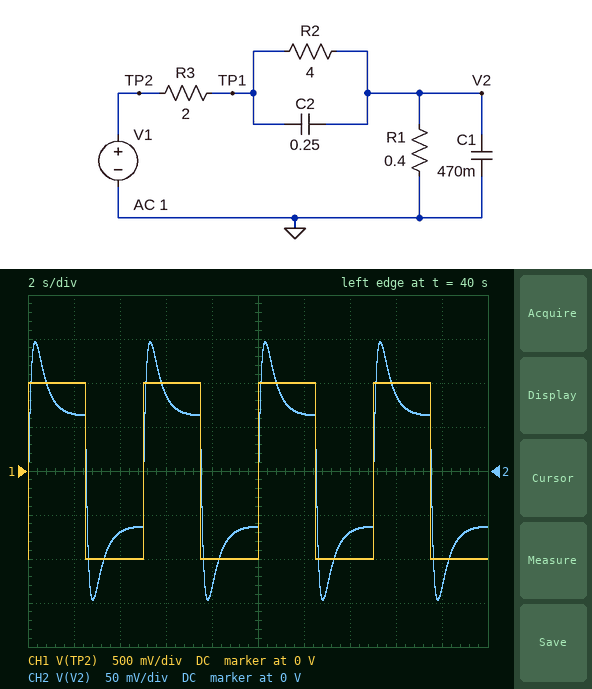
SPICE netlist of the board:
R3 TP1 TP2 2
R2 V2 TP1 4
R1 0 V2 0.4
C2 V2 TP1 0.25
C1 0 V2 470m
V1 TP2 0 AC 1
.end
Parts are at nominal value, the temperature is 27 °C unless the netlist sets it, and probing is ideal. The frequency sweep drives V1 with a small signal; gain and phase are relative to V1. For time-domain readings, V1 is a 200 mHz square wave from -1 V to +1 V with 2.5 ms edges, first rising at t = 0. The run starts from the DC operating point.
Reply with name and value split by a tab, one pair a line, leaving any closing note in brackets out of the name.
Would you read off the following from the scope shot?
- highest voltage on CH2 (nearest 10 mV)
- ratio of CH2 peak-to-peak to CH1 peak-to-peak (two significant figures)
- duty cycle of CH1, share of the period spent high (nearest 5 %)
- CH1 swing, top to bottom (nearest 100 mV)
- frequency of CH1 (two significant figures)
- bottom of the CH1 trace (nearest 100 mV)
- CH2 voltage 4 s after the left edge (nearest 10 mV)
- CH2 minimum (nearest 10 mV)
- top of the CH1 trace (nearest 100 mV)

highest voltage on CH2	150 mV
ratio of CH2 peak-to-peak to CH1 peak-to-peak	0.15
duty cycle of CH1, share of the period spent high	50 %
CH1 swing, top to bottom	2.0 V
frequency of CH1	200 mHz
bottom of the CH1 trace	-1.0 V
CH2 voltage 4 s after the left edge	-70 mV
CH2 minimum	-150 mV
top of the CH1 trace	1.0 V
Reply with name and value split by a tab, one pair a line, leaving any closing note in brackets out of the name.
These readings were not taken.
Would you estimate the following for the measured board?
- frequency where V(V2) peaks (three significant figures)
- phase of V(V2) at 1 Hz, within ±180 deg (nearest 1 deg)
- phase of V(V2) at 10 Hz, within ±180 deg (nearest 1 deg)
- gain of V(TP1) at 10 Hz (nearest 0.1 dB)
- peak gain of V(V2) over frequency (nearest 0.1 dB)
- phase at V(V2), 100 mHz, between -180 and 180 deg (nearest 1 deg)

frequency where V(V2) peaks	604 mHz
phase of V(V2) at 1 Hz, within ±180 deg	-30 deg
phase of V(V2) at 10 Hz, within ±180 deg	-82 deg
gain of V(TP1) at 10 Hz	-26.3 dB
peak gain of V(V2) over frequency	-18.6 dB
phase at V(V2), 100 mHz, between -180 and 180 deg	13 deg
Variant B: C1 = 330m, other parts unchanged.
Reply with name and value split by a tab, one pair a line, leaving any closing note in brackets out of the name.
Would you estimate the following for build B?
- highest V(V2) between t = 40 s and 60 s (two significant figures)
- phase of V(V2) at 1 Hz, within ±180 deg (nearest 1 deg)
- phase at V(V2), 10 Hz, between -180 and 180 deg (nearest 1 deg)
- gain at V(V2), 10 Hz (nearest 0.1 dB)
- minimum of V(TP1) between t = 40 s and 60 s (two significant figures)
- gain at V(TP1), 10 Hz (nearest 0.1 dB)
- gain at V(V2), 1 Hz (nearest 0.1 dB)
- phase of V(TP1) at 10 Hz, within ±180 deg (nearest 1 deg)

highest V(V2) between t = 40 s and 60 s	170 mV
phase of V(V2) at 1 Hz, within ±180 deg	-20 deg
phase at V(V2), 10 Hz, between -180 and 180 deg	-80 deg
gain at V(V2), 10 Hz	-32.5 dB
minimum of V(TP1) between t = 40 s and 60 s	-690 mV
gain at V(TP1), 10 Hz	-25.1 dB
gain at V(V2), 1 Hz	-18.1 dB
phase of V(TP1) at 10 Hz, within ±180 deg	-83 deg
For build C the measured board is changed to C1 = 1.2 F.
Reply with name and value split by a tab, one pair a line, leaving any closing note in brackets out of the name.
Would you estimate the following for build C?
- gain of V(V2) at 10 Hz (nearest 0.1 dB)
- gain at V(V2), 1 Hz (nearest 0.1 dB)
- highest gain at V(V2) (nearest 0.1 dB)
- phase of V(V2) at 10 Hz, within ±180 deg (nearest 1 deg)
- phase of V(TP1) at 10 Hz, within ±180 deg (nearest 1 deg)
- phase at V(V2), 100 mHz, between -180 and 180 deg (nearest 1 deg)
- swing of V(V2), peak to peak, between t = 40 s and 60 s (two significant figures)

gain of V(V2) at 10 Hz	-43.6 dB
gain at V(V2), 1 Hz	-25.1 dB
highest gain at V(V2)	-21.7 dB
phase of V(V2) at 10 Hz, within ±180 deg	-86 deg
phase of V(TP1) at 10 Hz, within ±180 deg	-87 deg
phase at V(V2), 100 mHz, between -180 and 180 deg	3 deg
swing of V(V2), peak to peak, between t = 40 s and 60 s	190 mV
